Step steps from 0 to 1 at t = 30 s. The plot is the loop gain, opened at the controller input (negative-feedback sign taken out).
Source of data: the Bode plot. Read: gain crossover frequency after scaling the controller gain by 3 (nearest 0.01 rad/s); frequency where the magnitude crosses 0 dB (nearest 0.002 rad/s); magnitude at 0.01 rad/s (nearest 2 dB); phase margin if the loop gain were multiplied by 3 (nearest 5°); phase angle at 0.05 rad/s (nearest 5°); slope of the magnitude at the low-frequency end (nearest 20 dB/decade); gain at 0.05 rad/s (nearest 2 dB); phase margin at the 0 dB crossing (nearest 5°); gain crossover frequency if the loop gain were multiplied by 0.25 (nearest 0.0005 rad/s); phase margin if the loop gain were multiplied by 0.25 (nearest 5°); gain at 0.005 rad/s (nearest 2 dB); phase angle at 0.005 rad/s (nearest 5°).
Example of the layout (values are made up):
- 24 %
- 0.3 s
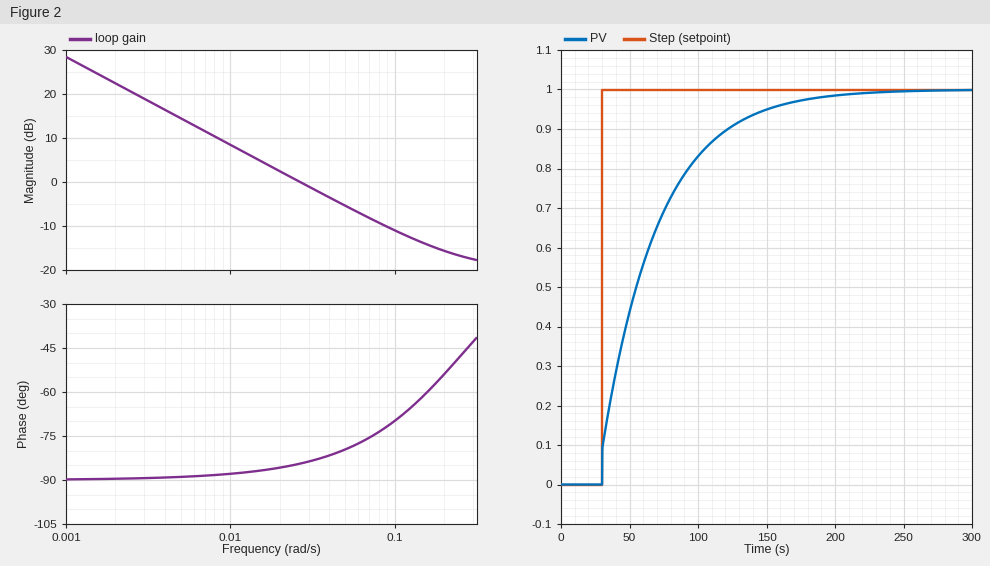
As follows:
- 0.08 rad/s
- 0.026 rad/s
- 8 dB
- 105°
- -80°
- -20 dB/decade
- -6 dB
- 95°
- 0.0065 rad/s
- 90°
- 14 dB
- -90°
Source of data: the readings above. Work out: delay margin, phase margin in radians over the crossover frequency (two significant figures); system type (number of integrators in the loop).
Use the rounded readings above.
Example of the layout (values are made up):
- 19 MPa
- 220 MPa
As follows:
- 64 s
- 1
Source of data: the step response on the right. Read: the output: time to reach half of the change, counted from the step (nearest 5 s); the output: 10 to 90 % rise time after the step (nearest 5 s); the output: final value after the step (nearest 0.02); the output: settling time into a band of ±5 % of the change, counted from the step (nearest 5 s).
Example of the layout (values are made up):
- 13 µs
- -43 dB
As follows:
- 25 s
- 90 s
- 1.00
- 120 s
